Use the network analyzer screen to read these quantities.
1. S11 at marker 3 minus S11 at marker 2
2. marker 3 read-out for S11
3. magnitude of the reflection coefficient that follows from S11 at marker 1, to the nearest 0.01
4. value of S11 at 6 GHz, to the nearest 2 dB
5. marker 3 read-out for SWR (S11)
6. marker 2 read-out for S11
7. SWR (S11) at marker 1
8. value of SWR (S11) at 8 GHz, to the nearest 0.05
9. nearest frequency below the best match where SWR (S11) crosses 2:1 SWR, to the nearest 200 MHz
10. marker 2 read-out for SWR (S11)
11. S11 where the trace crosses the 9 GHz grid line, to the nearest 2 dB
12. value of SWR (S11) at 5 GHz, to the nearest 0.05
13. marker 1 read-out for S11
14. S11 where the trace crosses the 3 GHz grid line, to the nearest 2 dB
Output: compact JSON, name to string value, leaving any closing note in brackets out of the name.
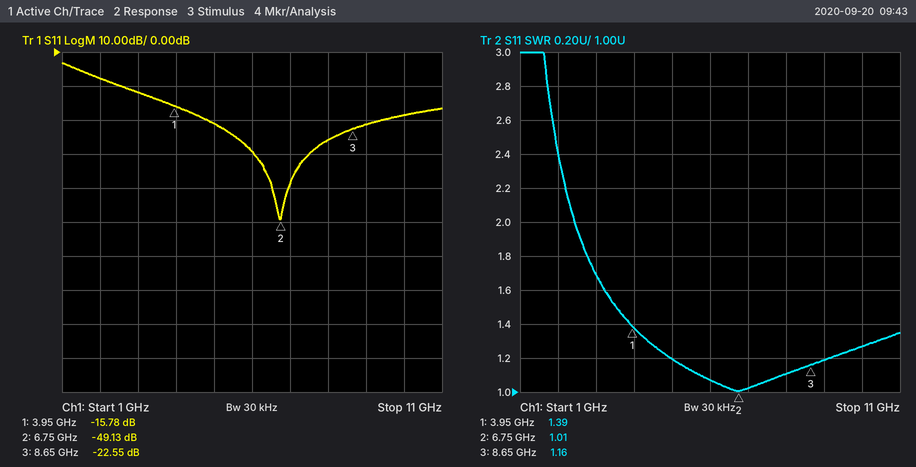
{"S11 at marker 3 minus S11 at marker 2": "26.58 dB", "marker 3 read-out for S11": "-22.55 dB", "magnitude of the reflection coefficient that follows from S11 at marker 1, to the nearest 0.01": "0.16", "value of S11 at 6 GHz, to the nearest 2 dB": "-30 dB", "marker 3 read-out for SWR": "1.16", "marker 2 read-out for S11": "-49.13 dB", "SWR (S11) at marker 1": "1.39", "value of SWR (S11) at 8 GHz, to the nearest 0.05": "1.10", "nearest frequency below the best match where SWR (S11) crosses 2:1 SWR, to the nearest 200 MHz": "2.4 GHz", "marker 2 read-out for SWR": "1.01", "S11 where the trace crosses the 9 GHz grid line, to the nearest 2 dB": "-22 dB", "value of SWR (S11) at 5 GHz, to the nearest 0.05": "1.20", "marker 1 read-out for S11": "-15.78 dB", "S11 where the trace crosses the 3 GHz grid line, to the nearest 2 dB": "-12 dB"}
